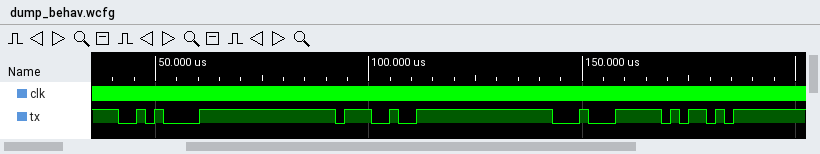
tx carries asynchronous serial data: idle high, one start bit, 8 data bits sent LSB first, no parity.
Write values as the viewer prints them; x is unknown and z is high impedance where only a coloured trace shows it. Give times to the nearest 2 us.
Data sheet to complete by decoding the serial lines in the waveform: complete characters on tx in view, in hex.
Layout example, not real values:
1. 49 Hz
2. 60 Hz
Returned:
1. 0A, 27, C4, AD
